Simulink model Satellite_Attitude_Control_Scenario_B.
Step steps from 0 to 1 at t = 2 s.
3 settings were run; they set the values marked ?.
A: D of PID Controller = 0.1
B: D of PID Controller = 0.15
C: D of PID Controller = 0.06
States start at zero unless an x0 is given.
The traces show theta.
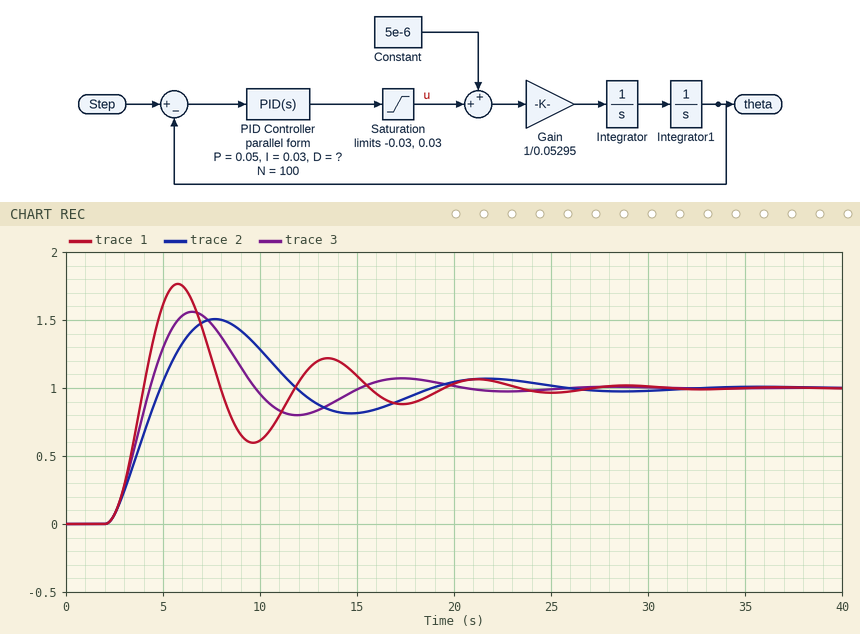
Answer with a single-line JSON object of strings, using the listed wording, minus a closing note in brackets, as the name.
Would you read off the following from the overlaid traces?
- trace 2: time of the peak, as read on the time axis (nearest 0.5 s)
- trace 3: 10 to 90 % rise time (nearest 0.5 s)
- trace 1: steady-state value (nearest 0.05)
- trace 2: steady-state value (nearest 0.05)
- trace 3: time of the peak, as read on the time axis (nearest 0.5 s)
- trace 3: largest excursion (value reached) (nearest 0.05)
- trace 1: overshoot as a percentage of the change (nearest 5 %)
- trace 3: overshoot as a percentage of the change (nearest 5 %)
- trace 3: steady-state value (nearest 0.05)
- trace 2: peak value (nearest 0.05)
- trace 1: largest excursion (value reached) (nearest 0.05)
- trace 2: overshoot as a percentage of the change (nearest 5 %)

{"trace 2: time of the peak, as read on the time axis": "7.5 s", "trace 3: 10 to 90 % rise time": "1.5 s", "trace 1: steady-state value": "1.00", "trace 2: steady-state value": "1.00", "trace 3: time of the peak, as read on the time axis": "6.5 s", "trace 3: largest excursion (value reached)": "1.55", "trace 1: overshoot as a percentage of the change": "75 %", "trace 3: overshoot as a percentage of the change": "55 %", "trace 3: steady-state value": "1.00", "trace 2: peak value": "1.50", "trace 1: largest excursion (value reached)": "1.75", "trace 2: overshoot as a percentage of the change": "50 %"}
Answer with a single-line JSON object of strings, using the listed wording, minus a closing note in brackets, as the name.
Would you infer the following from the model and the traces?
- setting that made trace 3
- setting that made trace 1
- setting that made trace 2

{"setting that made trace 3": "A", "setting that made trace 1": "C", "setting that made trace 2": "B"}
